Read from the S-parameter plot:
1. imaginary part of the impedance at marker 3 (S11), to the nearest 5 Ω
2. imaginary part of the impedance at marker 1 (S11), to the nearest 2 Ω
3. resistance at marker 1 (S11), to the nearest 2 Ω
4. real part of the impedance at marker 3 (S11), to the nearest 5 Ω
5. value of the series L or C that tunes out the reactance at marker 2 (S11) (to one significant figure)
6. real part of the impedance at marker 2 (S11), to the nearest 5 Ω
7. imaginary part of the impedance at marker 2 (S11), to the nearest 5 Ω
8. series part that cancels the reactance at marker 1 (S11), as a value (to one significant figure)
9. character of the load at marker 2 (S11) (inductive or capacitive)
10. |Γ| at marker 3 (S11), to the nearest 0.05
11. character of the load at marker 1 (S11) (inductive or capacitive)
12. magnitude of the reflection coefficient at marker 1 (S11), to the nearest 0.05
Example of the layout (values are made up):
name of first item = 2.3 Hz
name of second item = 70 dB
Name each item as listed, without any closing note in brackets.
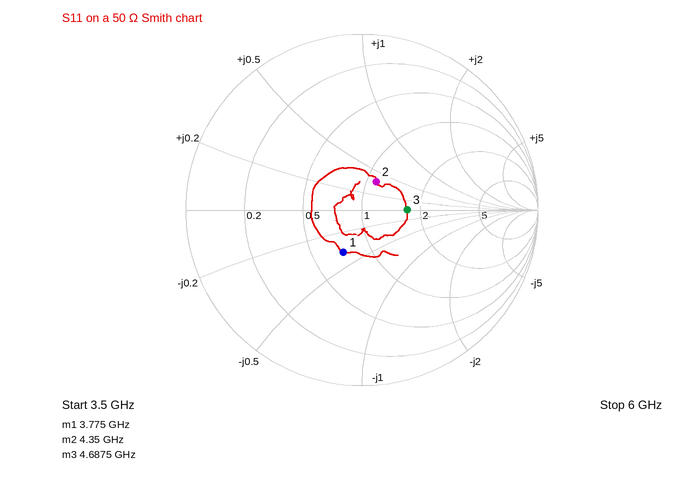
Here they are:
imaginary part of the impedance at marker 3 (S11), to the nearest 5 Ω = 0 Ω
imaginary part of the impedance at marker 1 (S11), to the nearest 2 Ω = -18 Ω
resistance at marker 1 (S11), to the nearest 2 Ω = 36 Ω
real part of the impedance at marker 3 (S11), to the nearest 5 Ω = 85 Ω
value of the series L or C that tunes out the reactance at marker 2 (S11) = 2 pF
real part of the impedance at marker 2 (S11), to the nearest 5 Ω = 55 Ω
imaginary part of the impedance at marker 2 (S11), to the nearest 5 Ω = +20 Ω
series part that cancels the reactance at marker 1 (S11), as a value = 800 pH
character of the load at marker 2 (S11) = inductive
|Γ| at marker 3 (S11), to the nearest 0.05 = 0.25
character of the load at marker 1 (S11) = capacitive
magnitude of the reflection coefficient at marker 1 (S11), to the nearest 0.05 = 0.25
